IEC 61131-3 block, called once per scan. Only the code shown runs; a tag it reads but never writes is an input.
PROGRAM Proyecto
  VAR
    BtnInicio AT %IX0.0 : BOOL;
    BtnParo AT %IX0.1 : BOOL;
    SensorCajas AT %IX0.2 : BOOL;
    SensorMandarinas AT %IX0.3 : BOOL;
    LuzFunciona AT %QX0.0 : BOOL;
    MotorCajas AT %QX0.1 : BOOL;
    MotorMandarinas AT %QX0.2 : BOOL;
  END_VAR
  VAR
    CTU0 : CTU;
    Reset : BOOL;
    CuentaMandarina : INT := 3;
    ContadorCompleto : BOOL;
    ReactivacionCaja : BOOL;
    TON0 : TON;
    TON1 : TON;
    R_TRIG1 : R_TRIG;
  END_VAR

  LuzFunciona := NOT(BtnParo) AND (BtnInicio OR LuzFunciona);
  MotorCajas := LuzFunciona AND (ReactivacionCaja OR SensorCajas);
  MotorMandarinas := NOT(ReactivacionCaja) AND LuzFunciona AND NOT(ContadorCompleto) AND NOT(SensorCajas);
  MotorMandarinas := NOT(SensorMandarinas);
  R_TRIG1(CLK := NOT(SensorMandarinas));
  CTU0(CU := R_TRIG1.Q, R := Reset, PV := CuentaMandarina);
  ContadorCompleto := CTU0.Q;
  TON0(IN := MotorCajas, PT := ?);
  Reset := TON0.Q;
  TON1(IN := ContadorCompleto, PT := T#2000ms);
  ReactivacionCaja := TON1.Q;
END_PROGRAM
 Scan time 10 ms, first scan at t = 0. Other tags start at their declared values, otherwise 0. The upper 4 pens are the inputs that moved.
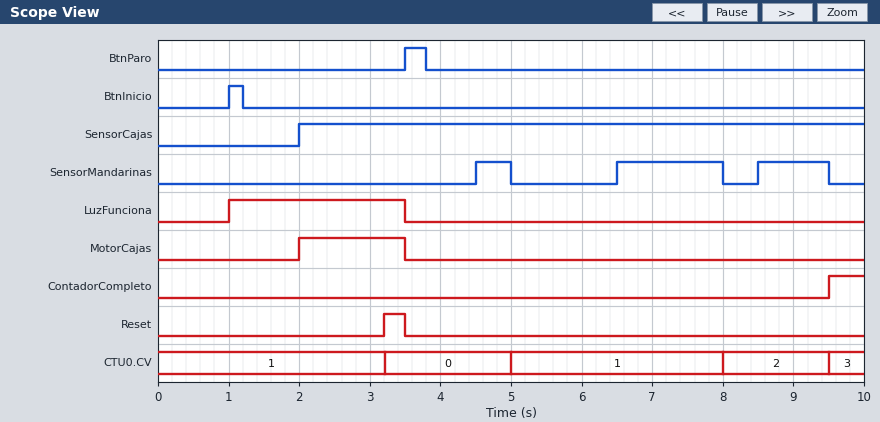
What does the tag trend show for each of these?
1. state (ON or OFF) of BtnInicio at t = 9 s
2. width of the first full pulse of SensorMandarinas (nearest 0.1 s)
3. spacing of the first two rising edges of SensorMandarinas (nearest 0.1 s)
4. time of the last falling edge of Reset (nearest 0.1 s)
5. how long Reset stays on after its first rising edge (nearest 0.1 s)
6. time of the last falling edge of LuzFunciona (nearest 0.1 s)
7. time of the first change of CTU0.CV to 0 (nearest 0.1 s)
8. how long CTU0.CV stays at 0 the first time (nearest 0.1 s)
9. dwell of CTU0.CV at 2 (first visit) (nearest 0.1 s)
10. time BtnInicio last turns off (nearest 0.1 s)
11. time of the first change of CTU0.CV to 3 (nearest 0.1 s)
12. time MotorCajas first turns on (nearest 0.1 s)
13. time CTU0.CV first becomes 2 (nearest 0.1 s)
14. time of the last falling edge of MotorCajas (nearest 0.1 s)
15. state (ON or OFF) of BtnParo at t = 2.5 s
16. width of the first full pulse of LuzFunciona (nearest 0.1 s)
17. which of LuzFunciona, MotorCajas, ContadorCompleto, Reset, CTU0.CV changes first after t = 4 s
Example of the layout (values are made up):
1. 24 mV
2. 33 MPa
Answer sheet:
1. OFF
2. 0.5 s
3. 2.0 s
4. 3.5 s
5. 0.3 s
6. 3.5 s
7. 3.2 s
8. 1.8 s
9. 1.5 s
10. 1.2 s
11. 9.5 s
12. 2.0 s
13. 8.0 s
14. 3.5 s
15. OFF
16. 2.5 s
17. CTU0.CV
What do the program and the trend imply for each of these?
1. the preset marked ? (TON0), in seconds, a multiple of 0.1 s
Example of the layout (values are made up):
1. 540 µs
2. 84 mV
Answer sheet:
1. 1.2 s
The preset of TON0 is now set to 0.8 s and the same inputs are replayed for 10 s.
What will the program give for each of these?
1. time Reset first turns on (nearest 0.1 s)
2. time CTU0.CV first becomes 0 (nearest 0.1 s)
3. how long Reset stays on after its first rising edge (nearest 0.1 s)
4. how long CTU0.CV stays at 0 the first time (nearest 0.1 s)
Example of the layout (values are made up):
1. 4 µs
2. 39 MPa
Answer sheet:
1. 2.8 s
2. 2.8 s
3. 0.7 s
4. 2.2 s
